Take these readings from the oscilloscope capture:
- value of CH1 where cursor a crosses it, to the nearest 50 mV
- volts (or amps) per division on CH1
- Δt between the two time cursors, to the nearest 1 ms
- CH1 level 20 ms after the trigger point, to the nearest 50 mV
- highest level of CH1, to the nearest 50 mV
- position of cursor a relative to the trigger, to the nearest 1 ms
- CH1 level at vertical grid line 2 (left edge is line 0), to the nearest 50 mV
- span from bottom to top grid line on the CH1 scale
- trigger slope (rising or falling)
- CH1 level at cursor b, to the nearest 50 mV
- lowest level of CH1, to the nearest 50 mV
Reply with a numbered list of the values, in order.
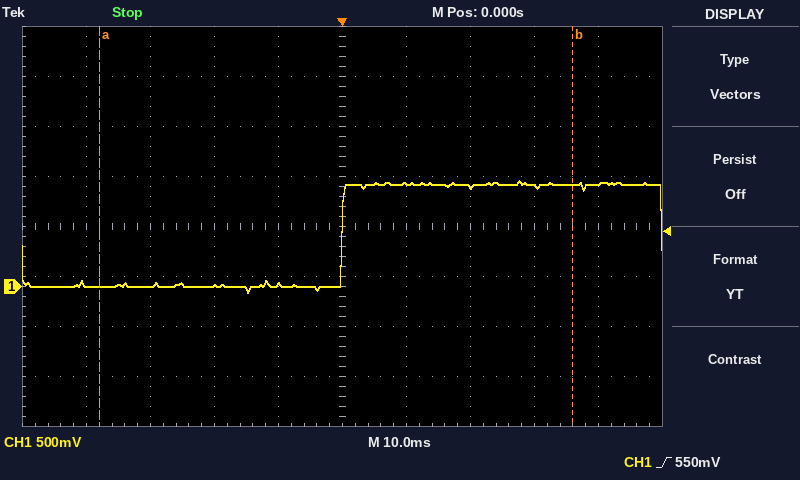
1. 0 mV
2. 500 mV
3. 74 ms
4. 1.00 V
5. 1.05 V
6. -38 ms
7. 0 mV
8. 4 V
9. rising
10. 1.00 V
11. -50 mV
